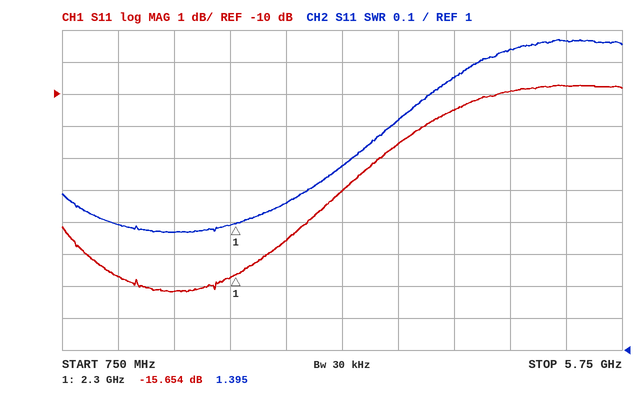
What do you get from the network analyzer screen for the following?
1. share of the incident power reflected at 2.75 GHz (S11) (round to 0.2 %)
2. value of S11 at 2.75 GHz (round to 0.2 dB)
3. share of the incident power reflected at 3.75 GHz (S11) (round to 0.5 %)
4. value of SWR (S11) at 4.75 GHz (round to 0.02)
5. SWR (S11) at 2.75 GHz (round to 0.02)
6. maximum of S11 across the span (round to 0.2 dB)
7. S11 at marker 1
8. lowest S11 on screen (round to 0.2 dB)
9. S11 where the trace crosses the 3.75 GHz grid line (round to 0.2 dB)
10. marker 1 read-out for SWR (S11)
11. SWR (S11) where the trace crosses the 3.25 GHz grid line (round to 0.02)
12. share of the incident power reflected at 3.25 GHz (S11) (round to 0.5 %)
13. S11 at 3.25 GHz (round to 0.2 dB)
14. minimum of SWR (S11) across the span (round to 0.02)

3.4 %
-14.6 dB
7.0 %
1.94
1.46
-9.8 dB
-15.654 dB
-16.2 dB
-11.6 dB
1.395
1.58
5.0 %
-13.0 dB
1.36
